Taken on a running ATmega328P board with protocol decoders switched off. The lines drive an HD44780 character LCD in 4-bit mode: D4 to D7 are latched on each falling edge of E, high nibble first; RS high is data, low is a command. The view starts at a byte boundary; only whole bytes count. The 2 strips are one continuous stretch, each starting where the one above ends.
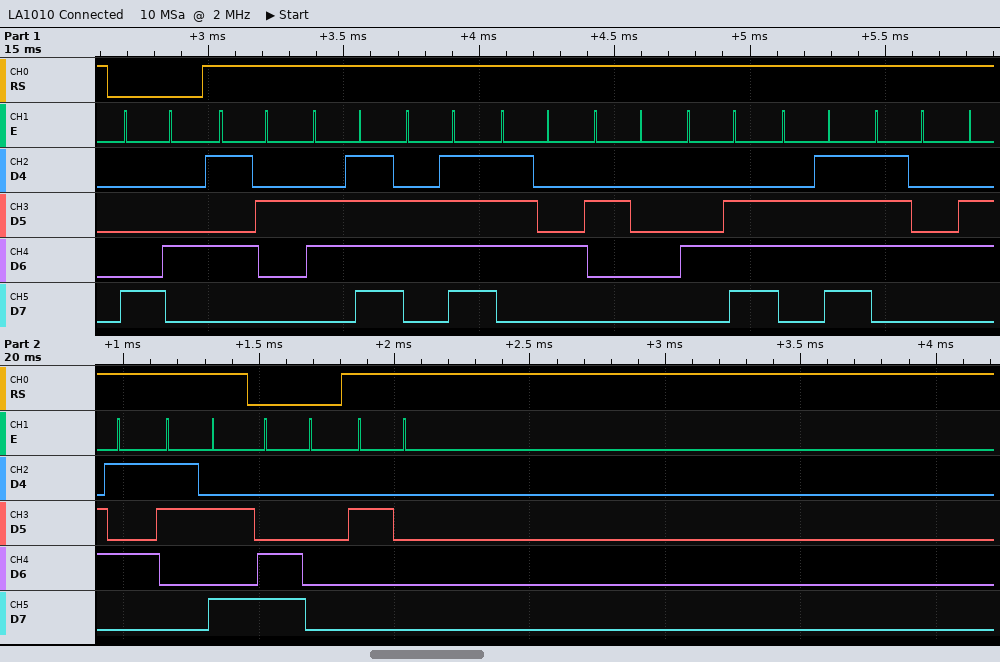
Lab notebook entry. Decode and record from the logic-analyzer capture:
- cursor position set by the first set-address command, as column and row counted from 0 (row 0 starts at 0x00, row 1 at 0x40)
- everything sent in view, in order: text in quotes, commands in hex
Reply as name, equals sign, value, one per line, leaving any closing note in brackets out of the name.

cursor position set by the first set-address command, as column and row counted from 0 = column 4, row 0
everything sent in view, in order: text in quotes, commands in hex = 0x84 "Root Note:" 0xC0 " "
